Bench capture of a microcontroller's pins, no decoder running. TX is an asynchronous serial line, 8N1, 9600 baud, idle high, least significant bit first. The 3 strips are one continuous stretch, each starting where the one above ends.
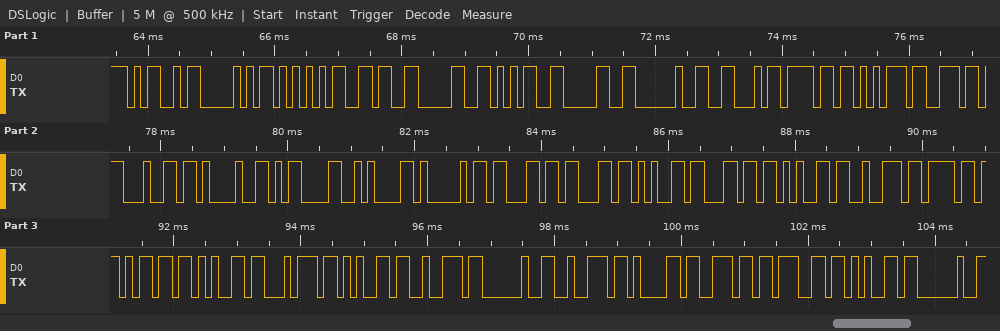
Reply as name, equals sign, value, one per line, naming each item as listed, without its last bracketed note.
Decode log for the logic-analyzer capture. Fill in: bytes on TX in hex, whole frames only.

bytes on TX in hex, whole frames only = 0x4D 0x50 0x55 0x36 0x30 0x35 0x30 0x20 0x46 0x6F 0x75 0x6E 0x64 0x21 0x0D 0x0A 0x41 0x63 0x63 0x65 0x6C 0x65 0x72 0x6F 0x6D 0x65 0x74 0x65 0x72 0x20 0x72 0x61 0x6E 0x67 0x65 0x20
